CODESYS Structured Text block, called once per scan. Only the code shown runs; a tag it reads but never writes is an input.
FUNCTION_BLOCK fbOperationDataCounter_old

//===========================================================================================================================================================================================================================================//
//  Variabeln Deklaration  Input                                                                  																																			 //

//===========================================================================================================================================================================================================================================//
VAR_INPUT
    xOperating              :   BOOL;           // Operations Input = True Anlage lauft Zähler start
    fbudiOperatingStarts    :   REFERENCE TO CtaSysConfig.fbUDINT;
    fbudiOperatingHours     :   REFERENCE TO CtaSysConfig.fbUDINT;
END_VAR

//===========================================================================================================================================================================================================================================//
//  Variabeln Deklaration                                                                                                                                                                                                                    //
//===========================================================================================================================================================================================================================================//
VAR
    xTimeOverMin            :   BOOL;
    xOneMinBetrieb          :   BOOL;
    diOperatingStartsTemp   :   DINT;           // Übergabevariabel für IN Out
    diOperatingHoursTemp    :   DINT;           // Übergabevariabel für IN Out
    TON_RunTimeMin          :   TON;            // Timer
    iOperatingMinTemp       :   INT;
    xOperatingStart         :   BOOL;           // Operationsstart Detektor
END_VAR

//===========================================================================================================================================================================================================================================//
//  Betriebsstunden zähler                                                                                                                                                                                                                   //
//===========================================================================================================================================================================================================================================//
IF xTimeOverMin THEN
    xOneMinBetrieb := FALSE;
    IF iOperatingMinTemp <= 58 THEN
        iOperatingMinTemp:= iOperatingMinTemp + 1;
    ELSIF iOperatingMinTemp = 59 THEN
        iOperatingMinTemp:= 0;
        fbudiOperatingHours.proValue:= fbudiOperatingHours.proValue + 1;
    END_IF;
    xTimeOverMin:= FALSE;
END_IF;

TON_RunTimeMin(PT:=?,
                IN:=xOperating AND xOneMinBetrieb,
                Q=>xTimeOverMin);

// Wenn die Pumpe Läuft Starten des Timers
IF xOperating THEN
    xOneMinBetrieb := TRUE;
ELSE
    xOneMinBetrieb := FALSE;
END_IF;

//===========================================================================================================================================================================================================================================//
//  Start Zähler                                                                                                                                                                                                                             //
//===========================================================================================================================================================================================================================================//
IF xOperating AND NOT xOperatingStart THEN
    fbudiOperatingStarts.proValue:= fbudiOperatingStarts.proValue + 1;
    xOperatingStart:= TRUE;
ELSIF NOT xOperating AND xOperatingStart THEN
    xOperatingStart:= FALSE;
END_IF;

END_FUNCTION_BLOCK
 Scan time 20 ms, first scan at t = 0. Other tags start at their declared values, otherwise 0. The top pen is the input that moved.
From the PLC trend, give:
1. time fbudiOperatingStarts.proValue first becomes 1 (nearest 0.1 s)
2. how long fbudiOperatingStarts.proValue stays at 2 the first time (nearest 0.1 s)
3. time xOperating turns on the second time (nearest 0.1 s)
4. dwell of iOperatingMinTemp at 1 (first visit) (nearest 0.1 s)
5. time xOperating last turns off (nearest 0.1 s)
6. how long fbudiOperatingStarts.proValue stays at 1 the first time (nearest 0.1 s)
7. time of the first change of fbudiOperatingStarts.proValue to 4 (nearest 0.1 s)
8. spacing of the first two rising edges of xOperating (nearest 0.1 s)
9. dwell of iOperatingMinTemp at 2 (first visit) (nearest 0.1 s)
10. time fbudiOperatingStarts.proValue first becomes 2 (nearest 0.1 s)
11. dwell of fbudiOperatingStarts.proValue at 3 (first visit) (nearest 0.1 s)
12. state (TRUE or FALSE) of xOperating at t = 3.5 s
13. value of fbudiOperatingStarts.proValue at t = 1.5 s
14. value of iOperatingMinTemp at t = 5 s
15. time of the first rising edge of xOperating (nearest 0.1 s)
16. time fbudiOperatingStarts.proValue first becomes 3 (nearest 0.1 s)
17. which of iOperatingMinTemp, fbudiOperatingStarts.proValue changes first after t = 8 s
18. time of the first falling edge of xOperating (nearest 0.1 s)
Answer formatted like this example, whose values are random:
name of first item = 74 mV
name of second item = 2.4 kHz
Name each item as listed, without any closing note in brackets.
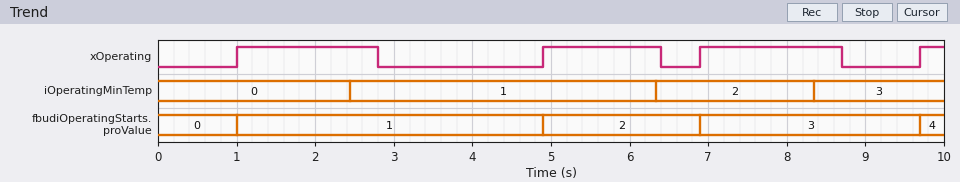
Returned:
time fbudiOperatingStarts.proValue first becomes 1 = 1.0 s
how long fbudiOperatingStarts.proValue stays at 2 the first time = 2.0 s
time xOperating turns on the second time = 4.9 s
dwell of iOperatingMinTemp at 1 (first visit) = 3.9 s
time xOperating last turns off = 8.7 s
how long fbudiOperatingStarts.proValue stays at 1 the first time = 3.9 s
time of the first change of fbudiOperatingStarts.proValue to 4 = 9.7 s
spacing of the first two rising edges of xOperating = 3.9 s
dwell of iOperatingMinTemp at 2 (first visit) = 2.0 s
time fbudiOperatingStarts.proValue first becomes 2 = 4.9 s
dwell of fbudiOperatingStarts.proValue at 3 (first visit) = 2.8 s
state (TRUE or FALSE) of xOperating at t = 3.5 s = FALSE
value of fbudiOperatingStarts.proValue at t = 1.5 s = 1
value of iOperatingMinTemp at t = 5 s = 1
time of the first rising edge of xOperating = 1.0 s
time fbudiOperatingStarts.proValue first becomes 3 = 6.9 s
which of iOperatingMinTemp, fbudiOperatingStarts.proValue changes first after t = 8 s = iOperatingMinTemp
time of the first falling edge of xOperating = 2.8 s
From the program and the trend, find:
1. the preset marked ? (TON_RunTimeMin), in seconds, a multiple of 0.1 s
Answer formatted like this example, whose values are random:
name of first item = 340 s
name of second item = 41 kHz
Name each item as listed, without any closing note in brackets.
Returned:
the preset marked ? (TON_RunTimeMin), in seconds, a multiple of 0.1 s = 1.4 s
